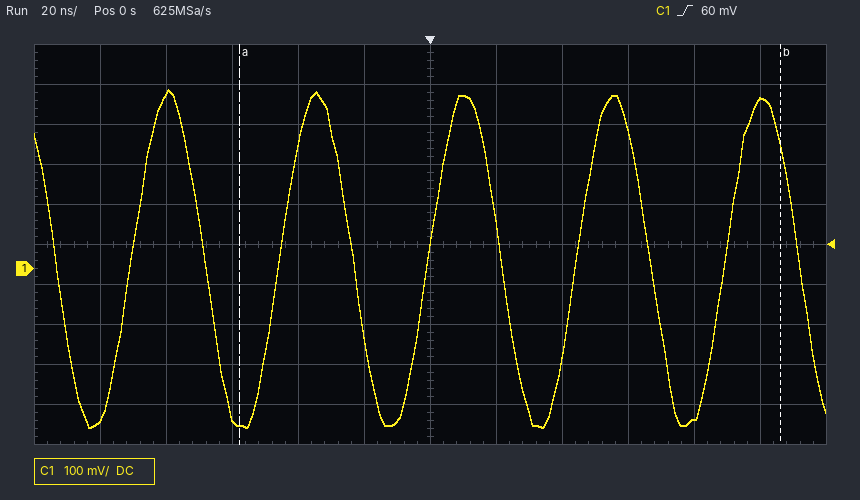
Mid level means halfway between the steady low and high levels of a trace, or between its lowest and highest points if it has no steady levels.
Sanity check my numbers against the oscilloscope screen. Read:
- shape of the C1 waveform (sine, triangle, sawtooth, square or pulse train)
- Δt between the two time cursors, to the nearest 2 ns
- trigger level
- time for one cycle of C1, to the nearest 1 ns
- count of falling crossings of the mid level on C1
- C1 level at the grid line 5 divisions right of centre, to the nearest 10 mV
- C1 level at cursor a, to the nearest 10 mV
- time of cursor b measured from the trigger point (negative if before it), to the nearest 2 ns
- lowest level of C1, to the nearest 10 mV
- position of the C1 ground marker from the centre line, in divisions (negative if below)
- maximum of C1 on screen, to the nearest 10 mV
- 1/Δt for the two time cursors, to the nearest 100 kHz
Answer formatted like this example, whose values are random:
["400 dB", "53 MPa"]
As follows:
["sine", "164 ns", "60 mV", "45 ns", "6", "420 mV", "-390 mV", "+106 ns", "-400 mV", "-0.6 div", "450 mV", "6.1 MHz"]
